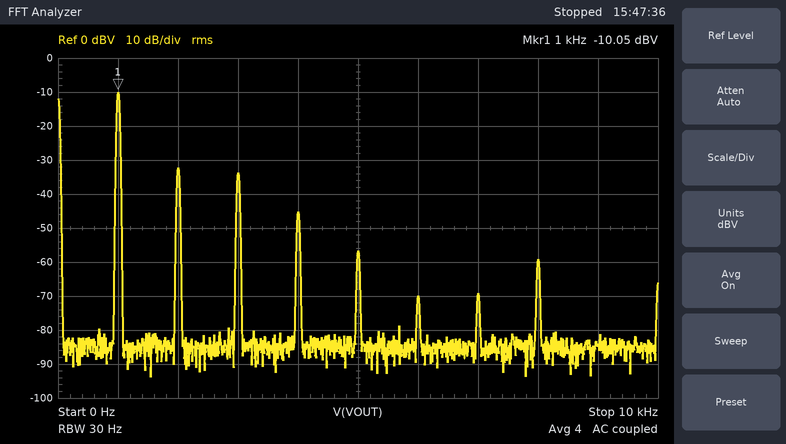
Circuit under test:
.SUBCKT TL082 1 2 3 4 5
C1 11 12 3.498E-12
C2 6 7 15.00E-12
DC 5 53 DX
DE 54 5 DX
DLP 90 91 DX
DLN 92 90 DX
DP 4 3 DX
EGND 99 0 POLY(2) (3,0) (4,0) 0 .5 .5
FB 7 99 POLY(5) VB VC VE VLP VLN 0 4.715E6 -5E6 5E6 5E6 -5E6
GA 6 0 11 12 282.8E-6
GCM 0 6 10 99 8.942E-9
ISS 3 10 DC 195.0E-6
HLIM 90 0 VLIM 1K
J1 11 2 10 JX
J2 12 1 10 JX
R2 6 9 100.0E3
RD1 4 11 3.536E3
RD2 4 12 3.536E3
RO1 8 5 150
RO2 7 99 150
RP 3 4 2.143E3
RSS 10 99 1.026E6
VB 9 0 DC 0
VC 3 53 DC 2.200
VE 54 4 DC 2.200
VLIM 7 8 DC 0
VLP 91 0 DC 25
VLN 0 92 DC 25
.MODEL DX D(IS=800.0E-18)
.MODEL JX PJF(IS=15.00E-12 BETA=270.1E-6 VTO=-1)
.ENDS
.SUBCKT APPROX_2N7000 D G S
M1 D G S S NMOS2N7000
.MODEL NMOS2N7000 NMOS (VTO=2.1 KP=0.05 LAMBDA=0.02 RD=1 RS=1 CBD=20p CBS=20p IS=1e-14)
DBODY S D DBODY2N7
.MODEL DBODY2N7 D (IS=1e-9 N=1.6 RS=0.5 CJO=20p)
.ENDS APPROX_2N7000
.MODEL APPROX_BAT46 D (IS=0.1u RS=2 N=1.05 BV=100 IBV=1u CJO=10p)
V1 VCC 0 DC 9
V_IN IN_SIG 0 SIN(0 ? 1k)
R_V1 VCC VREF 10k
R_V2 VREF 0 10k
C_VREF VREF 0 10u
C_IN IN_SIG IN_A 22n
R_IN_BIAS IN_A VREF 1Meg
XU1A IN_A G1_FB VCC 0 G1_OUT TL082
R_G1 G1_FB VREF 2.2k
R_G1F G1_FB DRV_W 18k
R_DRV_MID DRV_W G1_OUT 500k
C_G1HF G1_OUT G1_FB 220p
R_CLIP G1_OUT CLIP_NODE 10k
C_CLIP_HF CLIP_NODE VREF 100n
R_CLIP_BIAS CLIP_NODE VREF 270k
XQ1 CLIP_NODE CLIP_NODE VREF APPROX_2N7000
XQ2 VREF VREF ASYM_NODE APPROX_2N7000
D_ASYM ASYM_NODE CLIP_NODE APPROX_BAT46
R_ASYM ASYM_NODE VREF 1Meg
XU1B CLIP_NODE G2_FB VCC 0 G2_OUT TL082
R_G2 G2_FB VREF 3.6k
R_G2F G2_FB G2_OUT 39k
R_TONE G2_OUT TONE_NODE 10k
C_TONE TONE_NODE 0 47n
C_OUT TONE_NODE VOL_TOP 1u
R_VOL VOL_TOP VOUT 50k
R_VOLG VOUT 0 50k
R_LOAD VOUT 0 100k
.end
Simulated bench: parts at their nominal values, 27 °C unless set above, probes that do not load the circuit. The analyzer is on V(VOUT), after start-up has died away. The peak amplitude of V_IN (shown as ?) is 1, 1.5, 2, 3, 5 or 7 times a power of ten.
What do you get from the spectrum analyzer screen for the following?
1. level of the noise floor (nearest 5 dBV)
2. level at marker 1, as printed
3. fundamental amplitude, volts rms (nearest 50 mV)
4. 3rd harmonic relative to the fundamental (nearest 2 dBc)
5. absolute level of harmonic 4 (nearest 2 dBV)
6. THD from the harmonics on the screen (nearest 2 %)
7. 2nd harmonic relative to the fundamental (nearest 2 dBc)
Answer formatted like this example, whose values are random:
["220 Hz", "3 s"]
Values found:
["-85 dBV", "-10.05 dBV", "300 mV", "-24 dBc", "-46 dBV", "10 %", "-22 dBc"]
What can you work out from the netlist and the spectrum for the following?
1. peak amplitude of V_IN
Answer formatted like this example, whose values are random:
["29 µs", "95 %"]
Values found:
["30 mV"]
